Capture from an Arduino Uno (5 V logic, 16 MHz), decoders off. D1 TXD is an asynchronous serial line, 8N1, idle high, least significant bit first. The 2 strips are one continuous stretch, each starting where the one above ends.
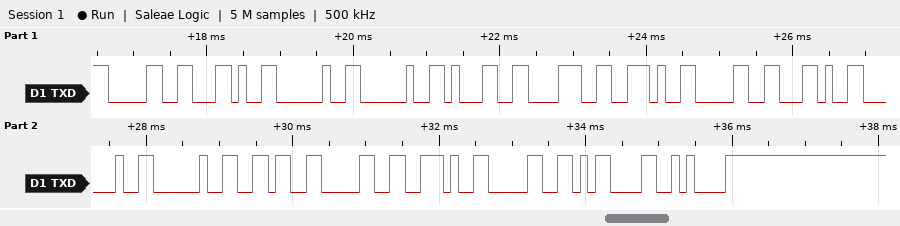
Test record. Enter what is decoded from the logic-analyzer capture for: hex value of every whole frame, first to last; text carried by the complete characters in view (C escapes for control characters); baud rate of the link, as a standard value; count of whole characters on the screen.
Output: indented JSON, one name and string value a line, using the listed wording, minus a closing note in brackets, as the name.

{
  "hex value of every whole frame, first to last": "30 2C 20 20 31 38 2E 30 2C 20 20 36 30 2E 30 0D 0A",
  "text carried by the complete characters in view": "\"0,  18.0,  60.0\\r\\n\"",
  "baud rate of the link, as a standard value": "9600 baud",
  "count of whole characters on the screen": "17"
}
